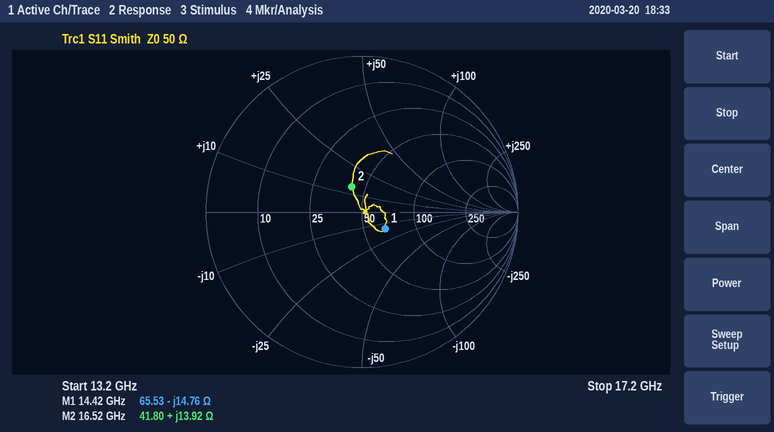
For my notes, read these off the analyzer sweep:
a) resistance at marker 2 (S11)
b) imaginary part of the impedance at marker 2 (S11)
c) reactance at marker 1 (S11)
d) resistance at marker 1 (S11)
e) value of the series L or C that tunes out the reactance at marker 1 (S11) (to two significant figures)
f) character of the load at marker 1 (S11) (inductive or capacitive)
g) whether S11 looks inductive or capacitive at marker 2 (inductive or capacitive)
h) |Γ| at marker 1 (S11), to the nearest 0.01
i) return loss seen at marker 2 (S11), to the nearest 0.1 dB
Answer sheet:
41.80 Ω
+13.92 Ω
-14.76 Ω
65.53 Ω
160 pH
capacitive
inductive
0.18
15.2 dB
